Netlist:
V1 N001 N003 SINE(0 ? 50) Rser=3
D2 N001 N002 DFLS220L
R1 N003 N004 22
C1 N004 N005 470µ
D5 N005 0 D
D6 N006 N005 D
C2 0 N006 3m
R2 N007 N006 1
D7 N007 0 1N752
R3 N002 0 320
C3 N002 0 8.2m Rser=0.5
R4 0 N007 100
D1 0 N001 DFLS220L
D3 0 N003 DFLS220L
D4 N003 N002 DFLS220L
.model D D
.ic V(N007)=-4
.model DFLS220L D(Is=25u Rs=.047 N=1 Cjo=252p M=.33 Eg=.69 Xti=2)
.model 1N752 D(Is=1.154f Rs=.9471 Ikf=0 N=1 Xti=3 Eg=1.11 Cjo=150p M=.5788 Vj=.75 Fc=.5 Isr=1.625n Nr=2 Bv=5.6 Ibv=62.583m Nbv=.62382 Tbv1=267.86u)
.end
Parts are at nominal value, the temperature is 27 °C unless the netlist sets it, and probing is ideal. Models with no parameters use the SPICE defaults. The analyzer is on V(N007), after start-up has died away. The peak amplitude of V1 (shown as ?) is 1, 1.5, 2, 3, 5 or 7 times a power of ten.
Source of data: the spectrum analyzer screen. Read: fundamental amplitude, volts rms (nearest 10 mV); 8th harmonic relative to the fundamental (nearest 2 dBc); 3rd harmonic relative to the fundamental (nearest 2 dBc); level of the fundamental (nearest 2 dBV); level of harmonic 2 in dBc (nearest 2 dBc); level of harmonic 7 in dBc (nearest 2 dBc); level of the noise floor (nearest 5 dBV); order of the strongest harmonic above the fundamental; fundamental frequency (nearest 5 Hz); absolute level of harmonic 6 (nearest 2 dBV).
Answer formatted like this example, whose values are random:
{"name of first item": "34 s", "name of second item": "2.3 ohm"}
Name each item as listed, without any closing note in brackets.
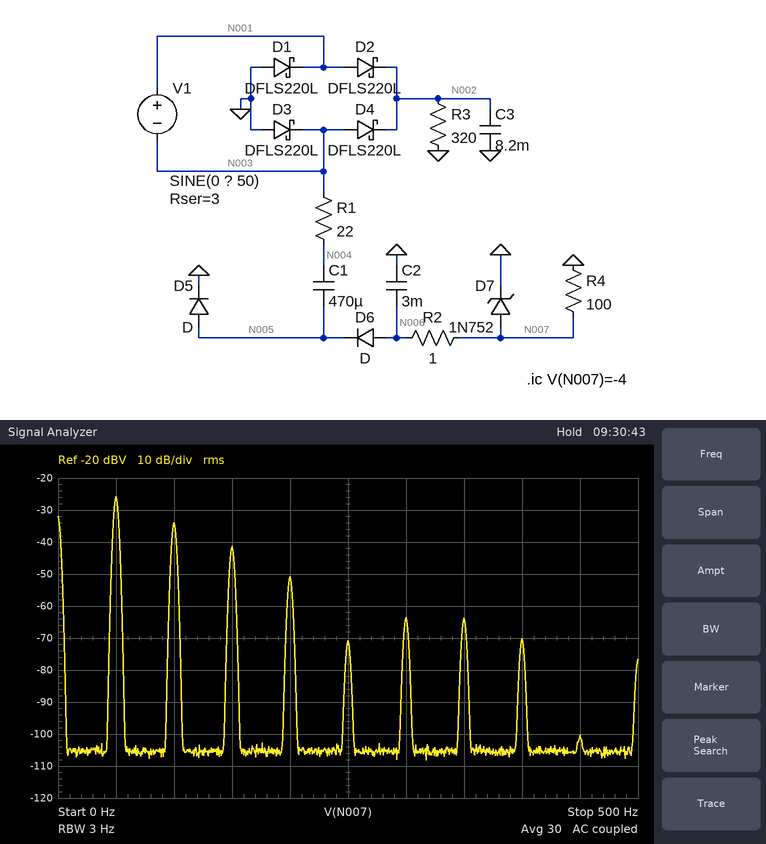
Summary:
{"fundamental amplitude, volts rms": "50 mV", "8th harmonic relative to the fundamental": "-44 dBc", "3rd harmonic relative to the fundamental": "-16 dBc", "level of the fundamental": "-26 dBV", "level of harmonic 2 in dBc": "-8 dBc", "level of harmonic 7 in dBc": "-38 dBc", "level of the noise floor": "-105 dBV", "order of the strongest harmonic above the fundamental": "2", "fundamental frequency": "50 Hz", "absolute level of harmonic 6": "-64 dBV"}
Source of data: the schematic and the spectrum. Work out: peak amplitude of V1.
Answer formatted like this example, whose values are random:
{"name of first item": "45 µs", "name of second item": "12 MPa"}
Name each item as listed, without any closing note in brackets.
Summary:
{"peak amplitude of V1": "15 V"}
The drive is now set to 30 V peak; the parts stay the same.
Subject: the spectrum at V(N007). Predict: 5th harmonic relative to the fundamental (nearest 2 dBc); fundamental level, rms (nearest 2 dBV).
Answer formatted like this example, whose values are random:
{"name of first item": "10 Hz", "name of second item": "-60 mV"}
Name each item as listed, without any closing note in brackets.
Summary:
{"5th harmonic relative to the fundamental": "-30 dBc", "fundamental level, rms": "-22 dBV"}
